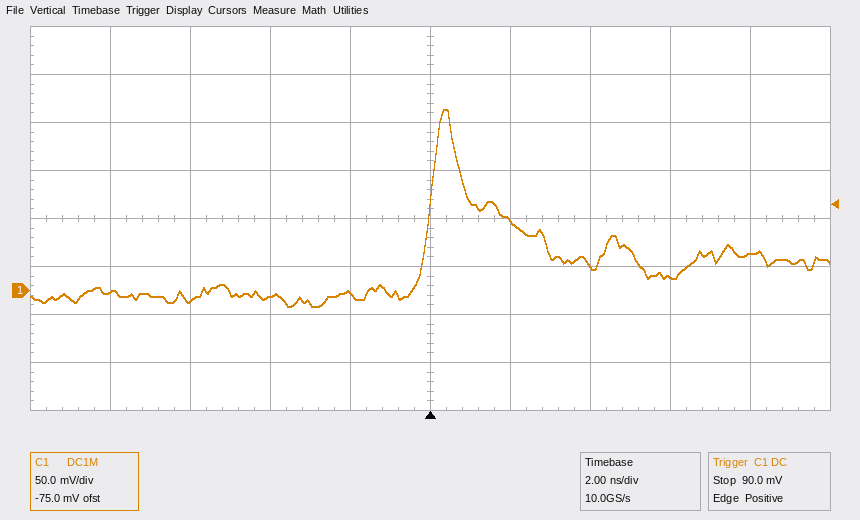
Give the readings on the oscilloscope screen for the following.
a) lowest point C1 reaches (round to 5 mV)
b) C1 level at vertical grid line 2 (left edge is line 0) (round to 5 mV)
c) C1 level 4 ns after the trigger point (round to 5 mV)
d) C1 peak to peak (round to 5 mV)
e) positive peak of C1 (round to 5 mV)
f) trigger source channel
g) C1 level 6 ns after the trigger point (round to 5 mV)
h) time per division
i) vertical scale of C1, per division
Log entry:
-15 mV
-10 mV
25 mV
205 mV
190 mV
C1
15 mV
2 ns
50 mV
